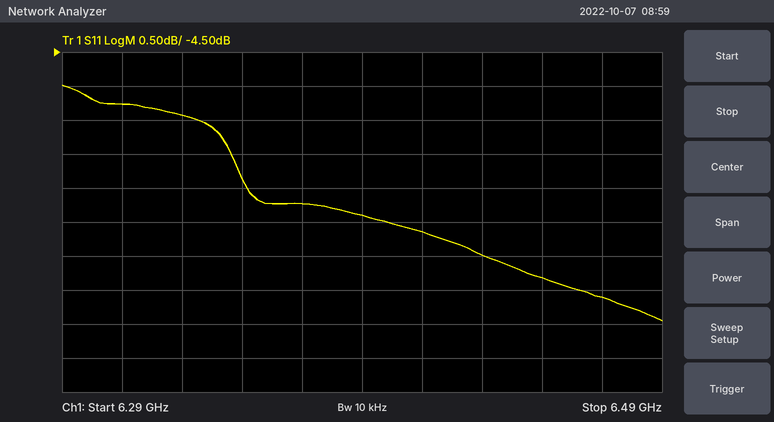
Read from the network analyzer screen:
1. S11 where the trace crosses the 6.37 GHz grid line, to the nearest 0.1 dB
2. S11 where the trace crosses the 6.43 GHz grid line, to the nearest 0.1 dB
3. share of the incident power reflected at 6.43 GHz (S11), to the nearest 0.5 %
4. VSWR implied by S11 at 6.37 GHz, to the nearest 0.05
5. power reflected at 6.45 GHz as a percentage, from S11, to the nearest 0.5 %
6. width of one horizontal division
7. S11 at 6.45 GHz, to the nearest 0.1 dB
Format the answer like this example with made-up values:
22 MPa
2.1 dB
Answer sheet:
-6.7 dB
-7.5 dB
18.0 %
2.70
16.5 %
20 MHz
-7.8 dB
